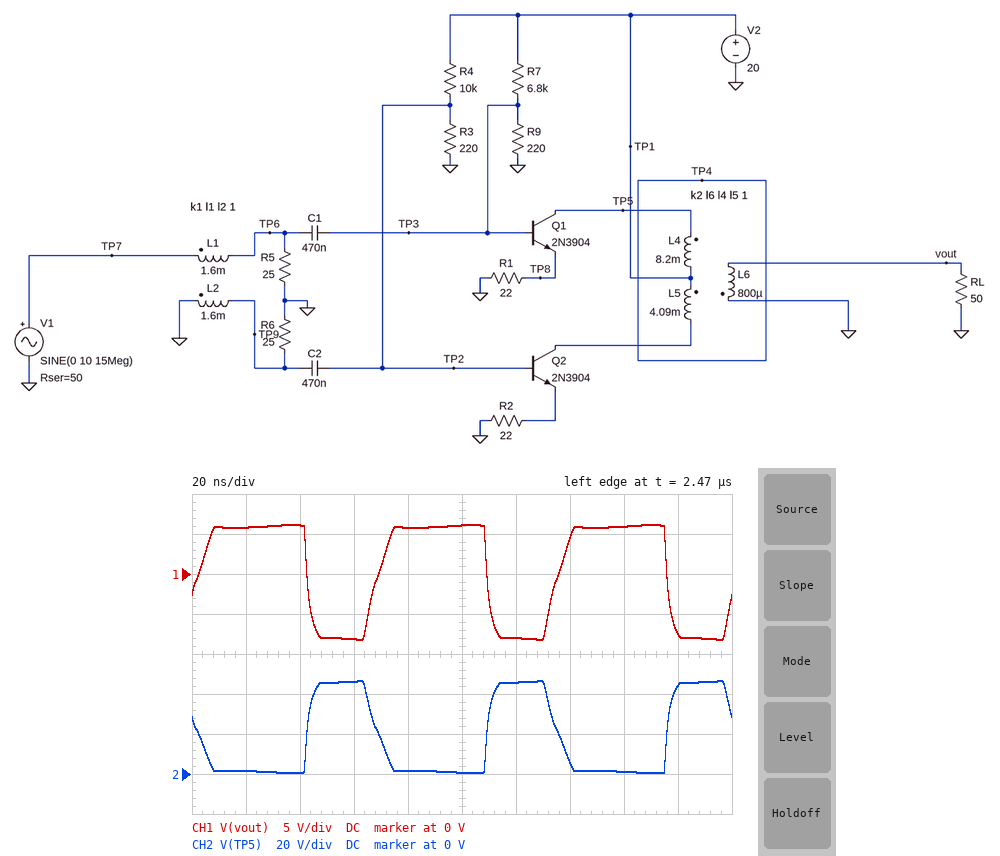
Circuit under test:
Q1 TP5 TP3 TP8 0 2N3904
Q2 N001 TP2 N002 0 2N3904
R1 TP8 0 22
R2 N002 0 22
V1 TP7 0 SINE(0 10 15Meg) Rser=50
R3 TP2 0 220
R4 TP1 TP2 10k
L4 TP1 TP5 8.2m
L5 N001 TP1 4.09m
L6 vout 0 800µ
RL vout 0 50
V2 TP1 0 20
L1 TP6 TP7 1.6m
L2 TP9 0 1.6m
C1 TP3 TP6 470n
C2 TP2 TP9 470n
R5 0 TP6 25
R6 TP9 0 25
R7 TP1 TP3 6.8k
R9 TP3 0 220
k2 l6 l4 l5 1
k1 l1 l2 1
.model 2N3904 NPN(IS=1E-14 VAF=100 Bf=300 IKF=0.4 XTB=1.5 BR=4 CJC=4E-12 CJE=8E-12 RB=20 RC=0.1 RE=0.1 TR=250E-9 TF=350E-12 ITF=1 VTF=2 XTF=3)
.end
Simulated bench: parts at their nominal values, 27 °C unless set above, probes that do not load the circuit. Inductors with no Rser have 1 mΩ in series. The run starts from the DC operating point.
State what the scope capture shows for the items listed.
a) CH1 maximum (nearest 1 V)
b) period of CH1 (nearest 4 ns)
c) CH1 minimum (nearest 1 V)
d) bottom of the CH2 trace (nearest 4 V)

6 V
68 ns
-8 V
0 V
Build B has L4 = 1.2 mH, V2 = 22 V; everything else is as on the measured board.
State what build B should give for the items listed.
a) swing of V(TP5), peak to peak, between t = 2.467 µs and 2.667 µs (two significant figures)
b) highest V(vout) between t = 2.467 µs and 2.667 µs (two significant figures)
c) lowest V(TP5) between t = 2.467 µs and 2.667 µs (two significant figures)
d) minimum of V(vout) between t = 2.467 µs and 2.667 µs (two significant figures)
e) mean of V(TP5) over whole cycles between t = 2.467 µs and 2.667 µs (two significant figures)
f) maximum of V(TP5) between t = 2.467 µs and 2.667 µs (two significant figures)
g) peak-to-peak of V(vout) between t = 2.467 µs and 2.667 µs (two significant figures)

19 V
6.3 V
14 V
-9.0 V
23 V
33 V
15 V
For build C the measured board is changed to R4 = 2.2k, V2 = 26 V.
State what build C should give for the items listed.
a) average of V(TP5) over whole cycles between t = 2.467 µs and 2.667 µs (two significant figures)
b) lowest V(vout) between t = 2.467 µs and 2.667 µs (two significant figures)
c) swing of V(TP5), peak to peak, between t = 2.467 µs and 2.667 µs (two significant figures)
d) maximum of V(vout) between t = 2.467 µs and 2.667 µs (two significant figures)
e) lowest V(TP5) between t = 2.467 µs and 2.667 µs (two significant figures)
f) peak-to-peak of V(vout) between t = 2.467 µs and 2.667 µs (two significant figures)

20 V
-10 V
58 V
7.9 V
700 mV
18 V
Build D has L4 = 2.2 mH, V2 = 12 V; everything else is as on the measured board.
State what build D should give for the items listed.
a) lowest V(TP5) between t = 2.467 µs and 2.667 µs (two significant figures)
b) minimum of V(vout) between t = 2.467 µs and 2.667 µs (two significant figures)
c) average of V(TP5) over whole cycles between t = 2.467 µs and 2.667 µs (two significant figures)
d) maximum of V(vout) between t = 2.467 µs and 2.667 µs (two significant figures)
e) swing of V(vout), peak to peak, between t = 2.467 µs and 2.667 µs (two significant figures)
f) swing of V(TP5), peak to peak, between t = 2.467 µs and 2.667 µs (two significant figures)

1.6 V
-5.1 V
12 V
6.3 V
11 V
19 V
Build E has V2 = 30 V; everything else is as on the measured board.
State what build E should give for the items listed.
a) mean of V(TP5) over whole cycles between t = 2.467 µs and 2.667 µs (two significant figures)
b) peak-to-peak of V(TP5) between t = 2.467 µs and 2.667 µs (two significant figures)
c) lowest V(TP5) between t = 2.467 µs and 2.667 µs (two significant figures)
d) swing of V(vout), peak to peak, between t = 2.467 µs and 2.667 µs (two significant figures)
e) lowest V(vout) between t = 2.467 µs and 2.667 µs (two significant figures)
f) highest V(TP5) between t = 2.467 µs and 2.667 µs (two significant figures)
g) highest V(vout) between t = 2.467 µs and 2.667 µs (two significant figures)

29 V
68 V
1.1 V
21 V
-12 V
69 V
9.0 V
